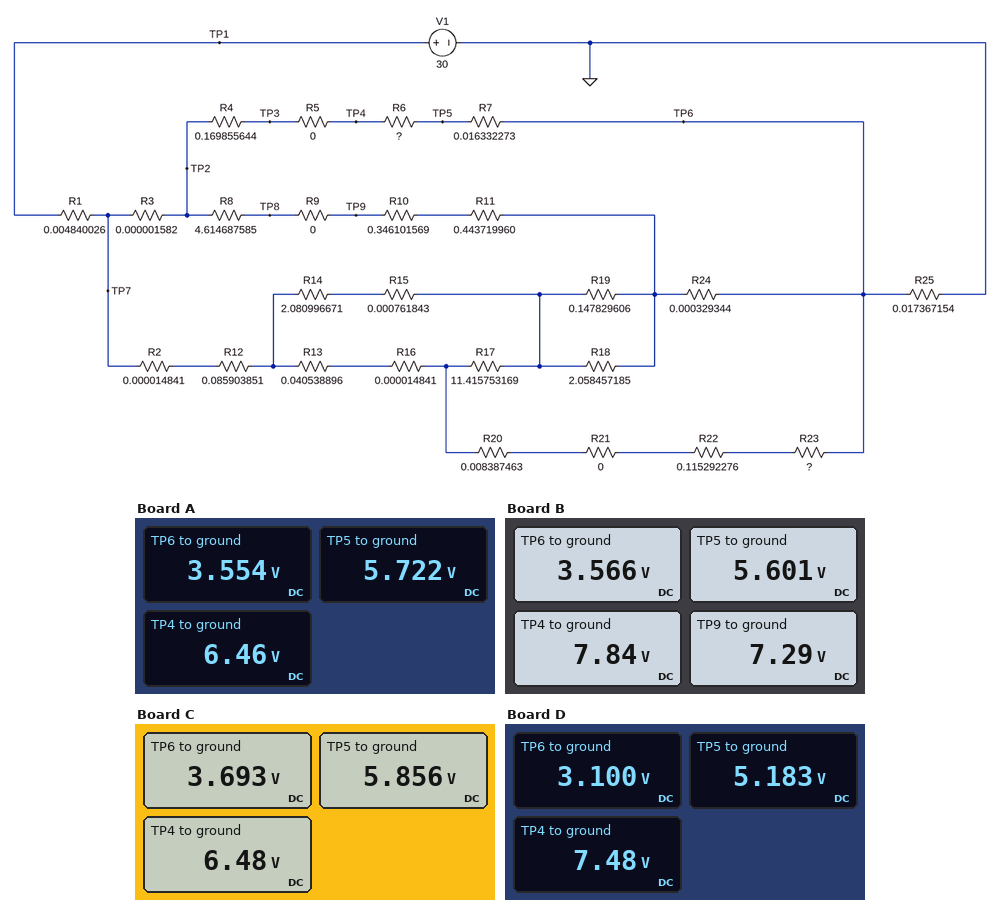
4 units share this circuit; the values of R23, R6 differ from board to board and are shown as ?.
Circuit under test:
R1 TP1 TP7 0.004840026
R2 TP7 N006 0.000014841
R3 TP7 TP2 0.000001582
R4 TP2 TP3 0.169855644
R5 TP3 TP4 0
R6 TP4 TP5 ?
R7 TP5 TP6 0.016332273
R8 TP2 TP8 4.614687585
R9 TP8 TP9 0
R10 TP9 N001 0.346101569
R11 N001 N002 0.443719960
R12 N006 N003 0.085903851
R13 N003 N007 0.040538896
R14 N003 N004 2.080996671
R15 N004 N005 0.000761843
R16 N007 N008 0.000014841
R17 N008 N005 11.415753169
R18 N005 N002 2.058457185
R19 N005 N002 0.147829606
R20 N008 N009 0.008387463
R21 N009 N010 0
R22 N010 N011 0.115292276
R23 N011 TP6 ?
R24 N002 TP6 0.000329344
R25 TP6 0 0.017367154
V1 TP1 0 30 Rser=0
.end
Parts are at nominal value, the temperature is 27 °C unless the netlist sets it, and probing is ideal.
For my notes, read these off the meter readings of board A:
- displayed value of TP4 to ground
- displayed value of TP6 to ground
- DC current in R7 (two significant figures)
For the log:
6.46 V
3.554 V
130 A
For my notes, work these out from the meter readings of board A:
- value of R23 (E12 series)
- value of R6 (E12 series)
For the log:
0.18 Ω
5.6 mΩ
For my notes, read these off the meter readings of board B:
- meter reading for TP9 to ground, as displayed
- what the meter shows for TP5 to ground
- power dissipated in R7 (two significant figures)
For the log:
7.29 V
5.601 V
250 W
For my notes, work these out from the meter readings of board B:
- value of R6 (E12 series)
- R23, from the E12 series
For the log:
0.018 Ω
0.12 Ω
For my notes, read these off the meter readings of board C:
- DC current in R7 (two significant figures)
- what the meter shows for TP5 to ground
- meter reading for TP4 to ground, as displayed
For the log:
130 A
5.856 V
6.48 V
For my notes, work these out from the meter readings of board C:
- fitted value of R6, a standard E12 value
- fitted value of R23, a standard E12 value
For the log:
4.7 mΩ
0.12 Ω
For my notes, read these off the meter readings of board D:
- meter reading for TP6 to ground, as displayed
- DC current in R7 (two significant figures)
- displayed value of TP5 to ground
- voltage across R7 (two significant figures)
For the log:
3.100 V
130 A
5.183 V
2.1 V
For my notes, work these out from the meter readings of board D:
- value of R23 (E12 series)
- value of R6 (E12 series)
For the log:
0.47 Ω
0.018 Ω
